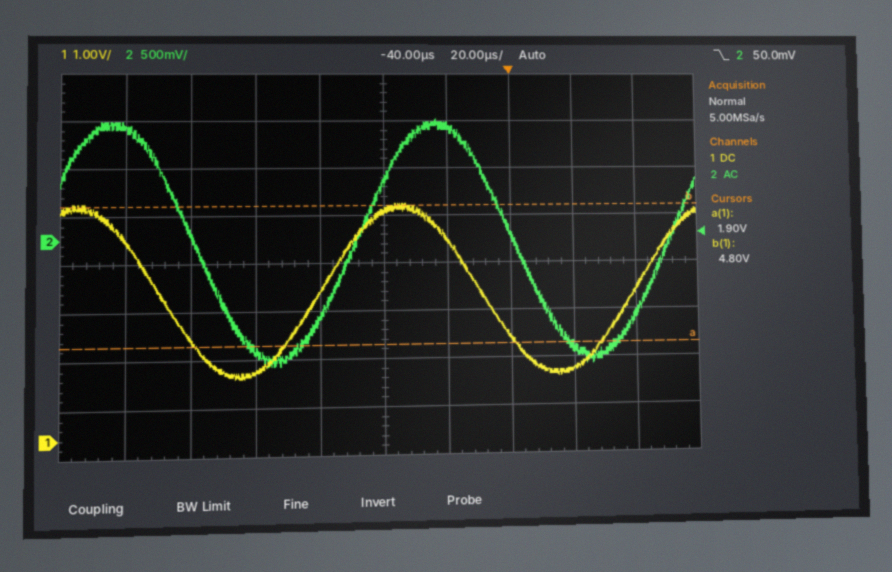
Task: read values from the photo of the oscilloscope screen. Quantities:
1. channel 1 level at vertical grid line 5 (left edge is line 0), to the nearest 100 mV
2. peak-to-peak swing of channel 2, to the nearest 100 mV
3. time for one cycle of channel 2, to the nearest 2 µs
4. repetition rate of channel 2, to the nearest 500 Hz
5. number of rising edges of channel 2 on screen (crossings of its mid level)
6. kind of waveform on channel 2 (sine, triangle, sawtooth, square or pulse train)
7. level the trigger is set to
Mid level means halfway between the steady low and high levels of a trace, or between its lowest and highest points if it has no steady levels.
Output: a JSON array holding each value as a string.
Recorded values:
["4.7 V", "2.60 V", "100 µs", "10.0 kHz", "2", "sine", "50.0 mV"]
